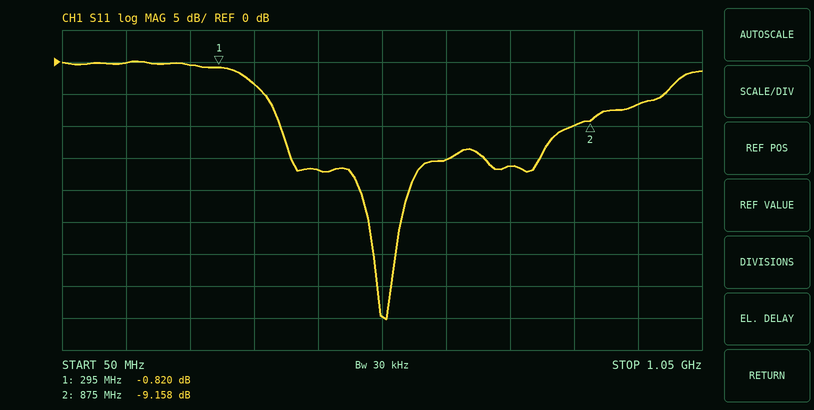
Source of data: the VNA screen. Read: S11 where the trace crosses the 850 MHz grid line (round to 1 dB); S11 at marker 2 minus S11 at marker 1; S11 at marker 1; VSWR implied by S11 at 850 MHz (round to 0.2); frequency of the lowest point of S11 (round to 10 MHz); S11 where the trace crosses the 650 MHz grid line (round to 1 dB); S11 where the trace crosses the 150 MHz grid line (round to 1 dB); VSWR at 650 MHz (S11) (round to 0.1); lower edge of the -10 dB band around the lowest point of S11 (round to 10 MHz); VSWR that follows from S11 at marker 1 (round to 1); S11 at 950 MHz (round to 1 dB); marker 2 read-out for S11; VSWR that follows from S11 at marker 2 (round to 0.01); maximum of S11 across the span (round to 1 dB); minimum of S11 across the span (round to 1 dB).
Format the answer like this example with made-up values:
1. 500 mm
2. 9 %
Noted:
1. -10 dB
2. -8.338 dB
3. -0.820 dB
4. 2.0
5. 560 MHz
6. -15 dB
7. 0 dB
8. 1.4
9. 390 MHz
10. 21
11. -7 dB
12. -9.158 dB
13. 2.07
14. 0 dB
15. -40 dB
